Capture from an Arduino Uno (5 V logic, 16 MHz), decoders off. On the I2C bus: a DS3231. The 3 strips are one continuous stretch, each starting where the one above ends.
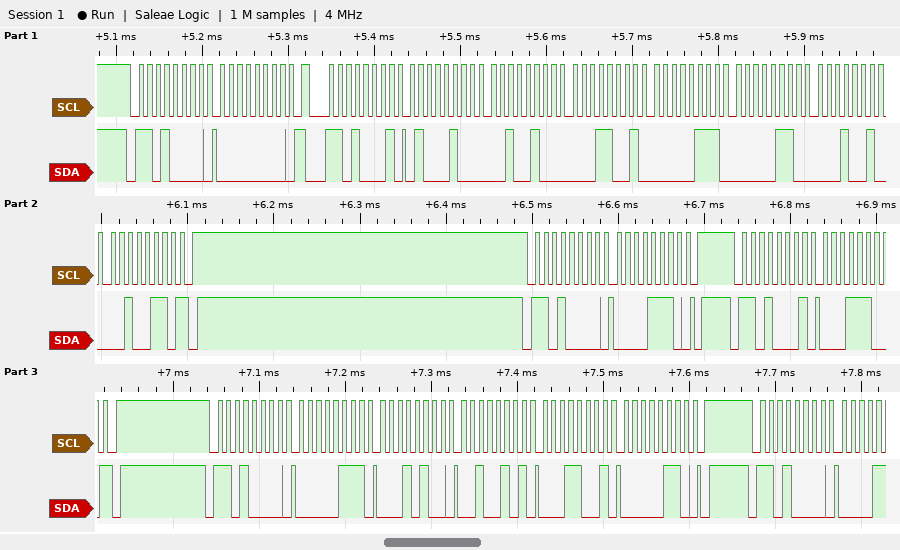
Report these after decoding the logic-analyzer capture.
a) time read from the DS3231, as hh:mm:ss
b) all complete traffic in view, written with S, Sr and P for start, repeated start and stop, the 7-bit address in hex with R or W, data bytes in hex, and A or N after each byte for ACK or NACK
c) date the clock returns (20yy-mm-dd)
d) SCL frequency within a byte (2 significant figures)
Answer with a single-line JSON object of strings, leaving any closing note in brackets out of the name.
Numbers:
{"time read from the DS3231, as hh:mm:ss": "19:24:44", "all complete traffic in view, written with S, Sr and P for start, repeated start and stop, the 7-bit address in hex with R or W, data bytes in hex, and A or N after each byte for ACK or NACK": "S 68W A 00 A Sr 68R A 44 A 24 A 19 A 07 A 06 A 12 A 26 N P S 68W A 0E A P S 68R A 1C N P S 68W A 07 A 14 A 25 A 19 A 06 A P S 68W A", "date the clock returns": "2026-12-06", "SCL frequency within a byte": "100 kHz"}
